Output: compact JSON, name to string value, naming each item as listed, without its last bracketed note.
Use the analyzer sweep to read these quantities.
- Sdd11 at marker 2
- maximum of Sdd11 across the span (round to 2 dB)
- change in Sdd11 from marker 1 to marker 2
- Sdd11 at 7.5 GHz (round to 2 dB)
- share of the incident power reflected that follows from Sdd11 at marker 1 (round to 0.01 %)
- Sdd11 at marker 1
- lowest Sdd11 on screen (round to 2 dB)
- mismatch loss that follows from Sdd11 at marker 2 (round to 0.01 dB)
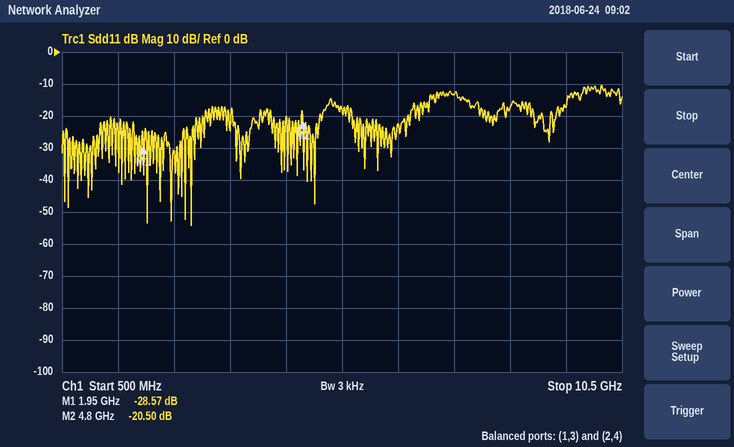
{"Sdd11 at marker 2": "-20.50 dB", "maximum of Sdd11 across the span": "-10 dB", "change in Sdd11 from marker 1 to marker 2": "8.07 dB", "Sdd11 at 7.5 GHz": "-14 dB", "share of the incident power reflected that follows from Sdd11 at marker 1": "0.14 %", "Sdd11 at marker 1": "-28.57 dB", "lowest Sdd11 on screen": "-54 dB", "mismatch loss that follows from Sdd11 at marker 2": "0.04 dB"}
